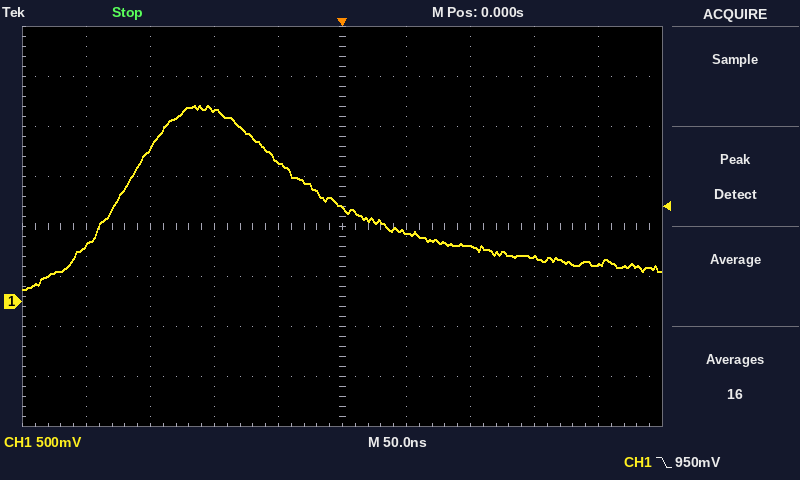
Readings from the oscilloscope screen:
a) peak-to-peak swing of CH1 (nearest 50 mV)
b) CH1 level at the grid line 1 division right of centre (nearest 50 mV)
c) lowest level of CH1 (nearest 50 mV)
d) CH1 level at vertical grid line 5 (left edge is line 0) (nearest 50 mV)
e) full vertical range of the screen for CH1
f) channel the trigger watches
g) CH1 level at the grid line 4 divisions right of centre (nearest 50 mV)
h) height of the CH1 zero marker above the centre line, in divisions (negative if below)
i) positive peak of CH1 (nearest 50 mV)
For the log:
1.85 V
700 mV
100 mV
950 mV
4 V
CH1
350 mV
-1.5 div
1.95 V
